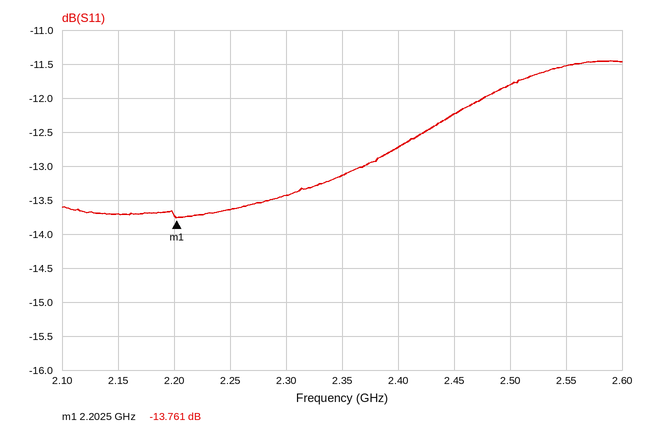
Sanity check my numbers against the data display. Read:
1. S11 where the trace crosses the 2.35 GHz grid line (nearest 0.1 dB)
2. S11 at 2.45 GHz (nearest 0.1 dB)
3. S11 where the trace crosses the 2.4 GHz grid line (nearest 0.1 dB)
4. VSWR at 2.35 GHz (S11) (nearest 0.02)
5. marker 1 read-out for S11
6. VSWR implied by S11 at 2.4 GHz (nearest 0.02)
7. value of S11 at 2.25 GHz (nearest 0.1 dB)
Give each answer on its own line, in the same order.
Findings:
-13.1 dB
-12.2 dB
-12.7 dB
1.56
-13.761 dB
1.60
-13.6 dB
